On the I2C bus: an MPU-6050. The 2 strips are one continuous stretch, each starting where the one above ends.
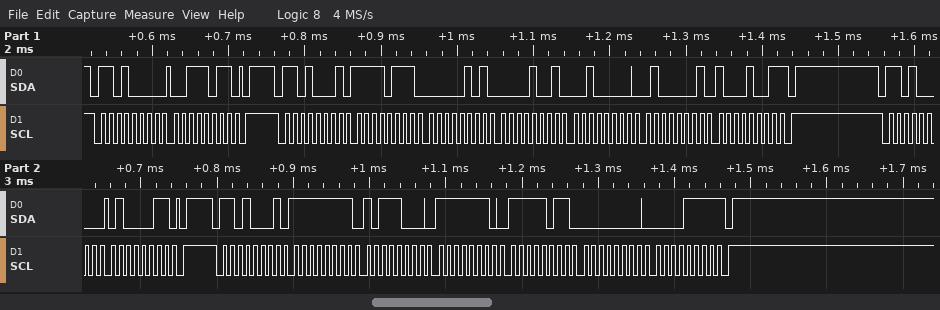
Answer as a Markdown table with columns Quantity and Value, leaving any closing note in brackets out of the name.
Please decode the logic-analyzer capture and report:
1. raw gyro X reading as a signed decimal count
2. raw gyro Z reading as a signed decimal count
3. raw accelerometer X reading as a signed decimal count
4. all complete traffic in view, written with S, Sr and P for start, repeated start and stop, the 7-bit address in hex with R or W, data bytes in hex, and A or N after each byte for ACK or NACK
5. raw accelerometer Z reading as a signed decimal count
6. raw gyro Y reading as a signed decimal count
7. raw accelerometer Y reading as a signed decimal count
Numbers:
| Quantity | Value |
|---|---|
| raw gyro X reading as a signed decimal count | -72 |
| raw gyro Z reading as a signed decimal count | 15 |
| raw accelerometer X reading as a signed decimal count | -2299 |
| all complete traffic in view, written with S, Sr and P for start, repeated start and stop, the 7-bit address in hex with R or W, data bytes in hex, and A or N after each byte for ACK or NACK | S 68W A 3B A P S 68R A F7 A 05 A 09 A 20 A 41 A 89 N P S 68W A 43 A P S 68R A FF A B8 A FE A FB A 00 A 0F N P |
| raw accelerometer Z reading as a signed decimal count | 16777 |
| raw gyro Y reading as a signed decimal count | -261 |
| raw accelerometer Y reading as a signed decimal count | 2336 |
